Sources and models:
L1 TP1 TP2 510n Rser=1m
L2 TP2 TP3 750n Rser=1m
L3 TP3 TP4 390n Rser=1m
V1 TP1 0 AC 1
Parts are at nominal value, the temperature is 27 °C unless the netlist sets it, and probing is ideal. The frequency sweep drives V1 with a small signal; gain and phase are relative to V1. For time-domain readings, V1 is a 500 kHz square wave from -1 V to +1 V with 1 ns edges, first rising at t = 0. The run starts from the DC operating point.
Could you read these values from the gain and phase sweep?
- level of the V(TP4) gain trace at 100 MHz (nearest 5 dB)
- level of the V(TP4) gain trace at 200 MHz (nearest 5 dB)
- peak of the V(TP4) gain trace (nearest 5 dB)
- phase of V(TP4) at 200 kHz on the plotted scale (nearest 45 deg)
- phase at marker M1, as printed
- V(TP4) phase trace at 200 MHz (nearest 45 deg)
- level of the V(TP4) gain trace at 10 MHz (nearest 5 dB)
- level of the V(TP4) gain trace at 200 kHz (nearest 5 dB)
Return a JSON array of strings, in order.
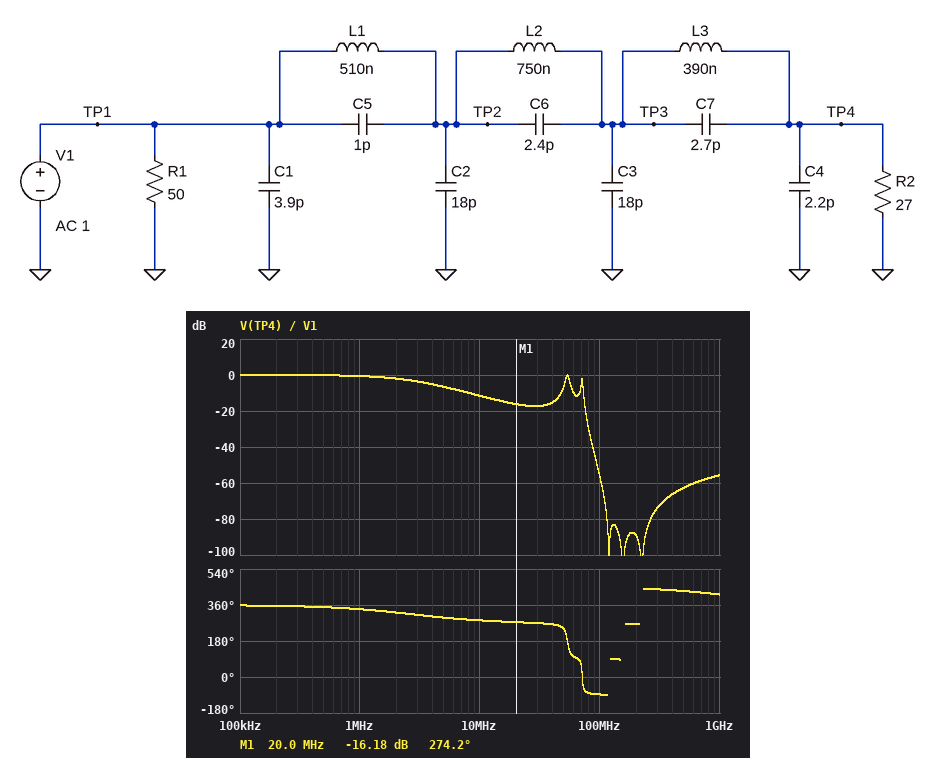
["-55 dB", "-90 dB", "0 dB", "360 deg", "274.2 deg", "270 deg", "-10 dB", "0 dB"]
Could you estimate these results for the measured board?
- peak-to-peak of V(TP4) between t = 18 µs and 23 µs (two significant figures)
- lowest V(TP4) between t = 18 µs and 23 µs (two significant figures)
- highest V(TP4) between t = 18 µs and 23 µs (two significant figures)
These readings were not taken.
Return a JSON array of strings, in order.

["2.0 V", "-1.0 V", "1.0 V"]
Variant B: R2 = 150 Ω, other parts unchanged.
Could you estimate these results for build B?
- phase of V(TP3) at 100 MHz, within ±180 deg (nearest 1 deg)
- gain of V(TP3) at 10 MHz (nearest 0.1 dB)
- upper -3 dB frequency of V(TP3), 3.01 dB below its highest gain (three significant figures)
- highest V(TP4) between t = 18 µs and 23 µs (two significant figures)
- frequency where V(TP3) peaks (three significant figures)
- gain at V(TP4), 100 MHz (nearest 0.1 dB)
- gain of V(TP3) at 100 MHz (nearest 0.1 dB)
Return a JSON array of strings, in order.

["6 deg", "-0.6 dB", "69.8 MHz", "1.2 V", "66.6 MHz", "-42.1 dB", "-33.1 dB"]
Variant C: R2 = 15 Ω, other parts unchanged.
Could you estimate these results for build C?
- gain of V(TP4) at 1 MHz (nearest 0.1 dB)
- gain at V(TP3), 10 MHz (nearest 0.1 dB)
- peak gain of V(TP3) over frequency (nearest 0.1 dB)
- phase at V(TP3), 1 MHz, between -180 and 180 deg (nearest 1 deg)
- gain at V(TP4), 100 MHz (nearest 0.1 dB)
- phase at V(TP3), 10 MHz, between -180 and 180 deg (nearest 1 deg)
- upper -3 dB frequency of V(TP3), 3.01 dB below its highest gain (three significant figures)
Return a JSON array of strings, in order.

["-1.7 dB", "-10.8 dB", "20.9 dB", "-25 deg", "-61.9 dB", "-24 deg", "71.7 MHz"]
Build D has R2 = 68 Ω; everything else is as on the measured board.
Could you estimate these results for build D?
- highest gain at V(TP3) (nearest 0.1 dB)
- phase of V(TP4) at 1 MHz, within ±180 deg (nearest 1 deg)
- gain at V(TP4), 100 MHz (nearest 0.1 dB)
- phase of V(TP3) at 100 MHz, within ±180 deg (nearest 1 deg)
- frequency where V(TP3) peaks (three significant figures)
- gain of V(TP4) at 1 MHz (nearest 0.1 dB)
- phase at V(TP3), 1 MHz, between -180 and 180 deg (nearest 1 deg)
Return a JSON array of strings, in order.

["9.2 dB", "-9 deg", "-48.8 dB", "3 deg", "69.9 MHz", "-0.1 dB", "-7 deg"]
